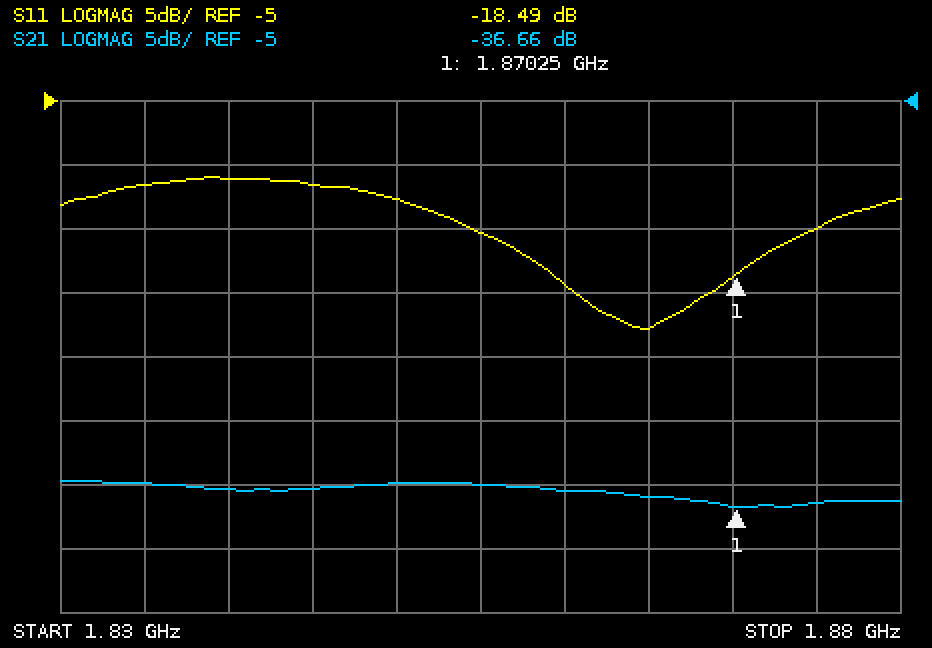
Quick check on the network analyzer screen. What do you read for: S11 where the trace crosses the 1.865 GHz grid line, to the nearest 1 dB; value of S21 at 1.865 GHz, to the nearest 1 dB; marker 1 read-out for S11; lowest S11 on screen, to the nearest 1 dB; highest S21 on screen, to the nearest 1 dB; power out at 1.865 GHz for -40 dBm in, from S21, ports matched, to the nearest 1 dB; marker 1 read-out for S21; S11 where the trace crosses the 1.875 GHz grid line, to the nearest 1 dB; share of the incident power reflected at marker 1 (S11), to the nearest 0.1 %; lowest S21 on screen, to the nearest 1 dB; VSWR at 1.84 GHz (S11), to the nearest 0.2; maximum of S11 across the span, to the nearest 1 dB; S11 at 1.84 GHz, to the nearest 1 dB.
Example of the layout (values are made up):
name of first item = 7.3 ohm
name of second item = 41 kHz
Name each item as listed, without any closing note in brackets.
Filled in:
S11 where the trace crosses the 1.865 GHz grid line, to the nearest 1 dB = -23 dB
value of S21 at 1.865 GHz, to the nearest 1 dB = -36 dB
marker 1 read-out for S11 = -18.49 dB
lowest S11 on screen, to the nearest 1 dB = -23 dB
highest S21 on screen, to the nearest 1 dB = -35 dB
power out at 1.865 GHz for -40 dBm in, from S21, ports matched, to the nearest 1 dB = -76 dBm
marker 1 read-out for S21 = -36.66 dB
S11 where the trace crosses the 1.875 GHz grid line, to the nearest 1 dB = -15 dB
share of the incident power reflected at marker 1 (S11), to the nearest 0.1 % = 1.4 %
lowest S21 on screen, to the nearest 1 dB = -37 dB
VSWR at 1.84 GHz (S11), to the nearest 0.2 = 1.8
maximum of S11 across the span, to the nearest 1 dB = -11 dB
S11 at 1.84 GHz, to the nearest 1 dB = -11 dB
